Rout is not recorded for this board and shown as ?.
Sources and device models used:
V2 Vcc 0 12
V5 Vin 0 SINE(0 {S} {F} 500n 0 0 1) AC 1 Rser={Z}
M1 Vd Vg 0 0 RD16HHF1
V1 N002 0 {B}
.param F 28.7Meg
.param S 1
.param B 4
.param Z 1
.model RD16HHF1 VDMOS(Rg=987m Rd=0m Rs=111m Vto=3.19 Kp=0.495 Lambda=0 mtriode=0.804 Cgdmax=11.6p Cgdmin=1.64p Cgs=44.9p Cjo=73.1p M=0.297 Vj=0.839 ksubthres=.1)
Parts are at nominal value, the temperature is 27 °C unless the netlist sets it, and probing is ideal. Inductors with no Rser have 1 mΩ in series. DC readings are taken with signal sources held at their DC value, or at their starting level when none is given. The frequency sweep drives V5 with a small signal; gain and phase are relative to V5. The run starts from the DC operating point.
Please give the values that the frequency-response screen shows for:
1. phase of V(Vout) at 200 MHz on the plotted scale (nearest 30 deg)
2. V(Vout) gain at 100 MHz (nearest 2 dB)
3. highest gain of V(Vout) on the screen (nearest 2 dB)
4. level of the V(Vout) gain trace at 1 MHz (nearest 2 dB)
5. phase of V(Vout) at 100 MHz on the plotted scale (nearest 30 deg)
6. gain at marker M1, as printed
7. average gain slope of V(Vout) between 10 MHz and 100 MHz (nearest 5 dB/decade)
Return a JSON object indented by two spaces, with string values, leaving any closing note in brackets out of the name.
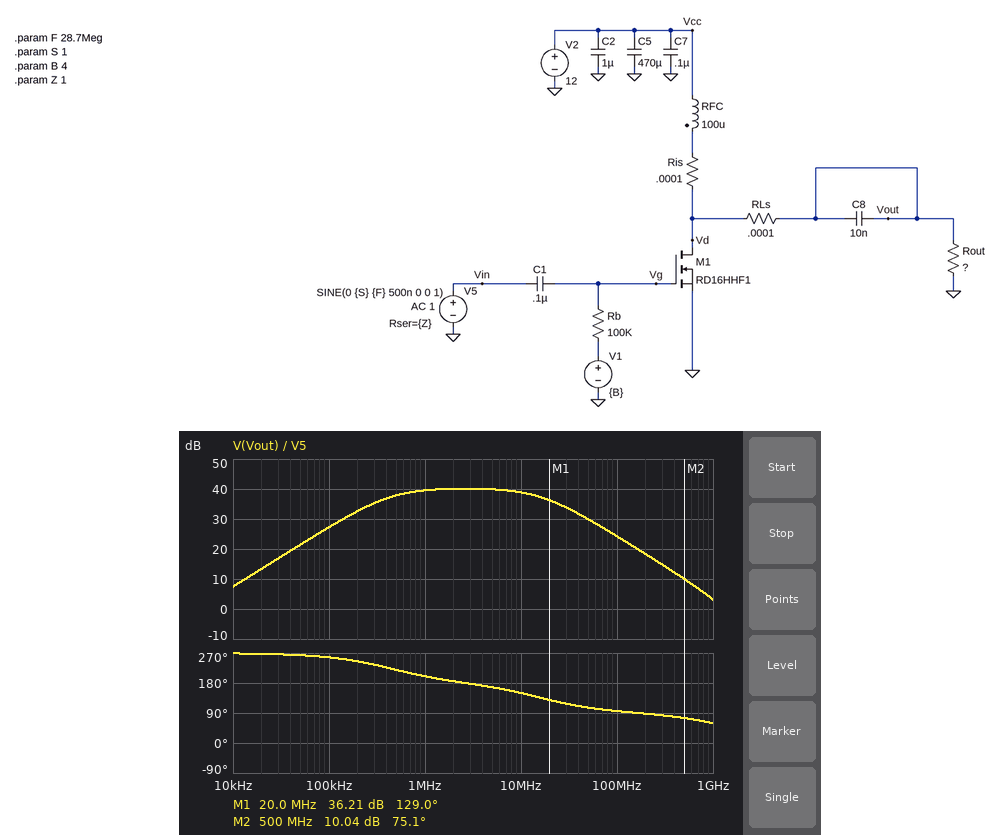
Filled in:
{
  "phase of V(Vout) at 200 MHz on the plotted scale": "90 deg",
  "V(Vout) gain at 100 MHz": "24 dB",
  "highest gain of V(Vout) on the screen": "40 dB",
  "level of the V(Vout) gain trace at 1 MHz": "40 dB",
  "phase of V(Vout) at 100 MHz on the plotted scale": "90 deg",
  "gain at marker M1, as printed": "36.21 dB",
  "average gain slope of V(Vout) between 10 MHz and 100 MHz": "-15 dB/decade"
}
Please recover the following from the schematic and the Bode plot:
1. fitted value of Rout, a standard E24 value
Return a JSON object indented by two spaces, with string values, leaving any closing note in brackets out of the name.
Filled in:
{
  "fitted value of Rout, a standard E24 value": "270 Ω"
}
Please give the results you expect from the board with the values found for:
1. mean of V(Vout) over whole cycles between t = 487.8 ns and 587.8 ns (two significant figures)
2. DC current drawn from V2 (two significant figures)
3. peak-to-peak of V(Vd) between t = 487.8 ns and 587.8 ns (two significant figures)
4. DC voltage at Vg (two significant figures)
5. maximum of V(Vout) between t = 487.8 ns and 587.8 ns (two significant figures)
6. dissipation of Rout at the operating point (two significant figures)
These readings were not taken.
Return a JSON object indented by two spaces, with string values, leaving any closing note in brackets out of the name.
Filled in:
{
  "mean of V(Vout) over whole cycles between t = 487.8 ns and 587.8 ns": "11 V",
  "DC current drawn from V2": "200 mA",
  "peak-to-peak of V(Vd) between t = 487.8 ns and 587.8 ns": "43 V",
  "DC voltage at Vg": "4.0 V",
  "maximum of V(Vout) between t = 487.8 ns and 587.8 ns": "43 V",
  "dissipation of Rout at the operating point": "530 mW"
}
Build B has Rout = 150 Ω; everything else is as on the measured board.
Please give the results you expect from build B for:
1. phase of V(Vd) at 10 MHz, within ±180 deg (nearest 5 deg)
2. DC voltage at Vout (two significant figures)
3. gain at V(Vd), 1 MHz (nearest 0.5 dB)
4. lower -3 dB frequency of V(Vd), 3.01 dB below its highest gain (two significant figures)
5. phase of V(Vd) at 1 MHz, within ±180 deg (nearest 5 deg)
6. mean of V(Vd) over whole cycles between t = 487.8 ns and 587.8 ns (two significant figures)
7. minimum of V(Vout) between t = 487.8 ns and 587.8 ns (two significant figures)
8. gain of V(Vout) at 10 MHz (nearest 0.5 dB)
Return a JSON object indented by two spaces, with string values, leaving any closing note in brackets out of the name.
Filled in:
{
  "phase of V(Vd) at 10 MHz, within ±180 deg": "160 deg",
  "DC voltage at Vout": "12 V",
  "gain at V(Vd), 1 MHz": "35.0 dB",
  "lower -3 dB frequency of V(Vd), 3.01 dB below its highest gain": "240 kHz",
  "phase of V(Vd) at 1 MHz, within ±180 deg": "-170 deg",
  "mean of V(Vd) over whole cycles between t = 487.8 ns and 587.8 ns": "10 V",
  "minimum of V(Vout) between t = 487.8 ns and 587.8 ns": "380 mV",
  "gain of V(Vout) at 10 MHz": "34.5 dB"
}
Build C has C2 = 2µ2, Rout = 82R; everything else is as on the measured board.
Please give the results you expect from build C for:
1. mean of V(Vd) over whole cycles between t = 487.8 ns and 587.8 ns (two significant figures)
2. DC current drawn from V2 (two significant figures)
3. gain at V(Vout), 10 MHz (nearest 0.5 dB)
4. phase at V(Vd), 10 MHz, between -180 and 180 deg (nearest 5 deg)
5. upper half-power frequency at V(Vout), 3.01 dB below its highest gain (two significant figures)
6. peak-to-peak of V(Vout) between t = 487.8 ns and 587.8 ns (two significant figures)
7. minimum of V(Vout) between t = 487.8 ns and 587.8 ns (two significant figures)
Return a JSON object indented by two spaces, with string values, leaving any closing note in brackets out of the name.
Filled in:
{
  "mean of V(Vd) over whole cycles between t = 487.8 ns and 587.8 ns": "9.2 V",
  "DC current drawn from V2": "300 mA",
  "gain at V(Vout), 10 MHz": "29.5 dB",
  "phase at V(Vd), 10 MHz, between -180 and 180 deg": "170 deg",
  "upper half-power frequency at V(Vout), 3.01 dB below its highest gain": "54 MHz",
  "peak-to-peak of V(Vout) between t = 487.8 ns and 587.8 ns": "24 V",
  "minimum of V(Vout) between t = 487.8 ns and 587.8 ns": "500 mV"
}
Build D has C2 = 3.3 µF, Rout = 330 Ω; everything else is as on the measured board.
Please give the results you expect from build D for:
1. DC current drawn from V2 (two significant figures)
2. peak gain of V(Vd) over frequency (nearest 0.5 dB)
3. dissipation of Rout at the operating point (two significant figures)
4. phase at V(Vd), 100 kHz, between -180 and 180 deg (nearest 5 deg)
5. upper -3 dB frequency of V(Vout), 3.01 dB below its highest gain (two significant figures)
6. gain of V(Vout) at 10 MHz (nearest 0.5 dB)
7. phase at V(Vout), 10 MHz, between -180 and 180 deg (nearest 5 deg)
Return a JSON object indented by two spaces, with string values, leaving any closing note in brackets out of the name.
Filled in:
{
  "DC current drawn from V2": "190 mA",
  "peak gain of V(Vd) over frequency": "42.0 dB",
  "dissipation of Rout at the operating point": "440 mW",
  "phase at V(Vd), 100 kHz, between -180 and 180 deg": "-100 deg",
  "upper -3 dB frequency of V(Vout), 3.01 dB below its highest gain": "14 MHz",
  "gain of V(Vout) at 10 MHz": "40.0 dB",
  "phase at V(Vout), 10 MHz, between -180 and 180 deg": "145 deg"
}
